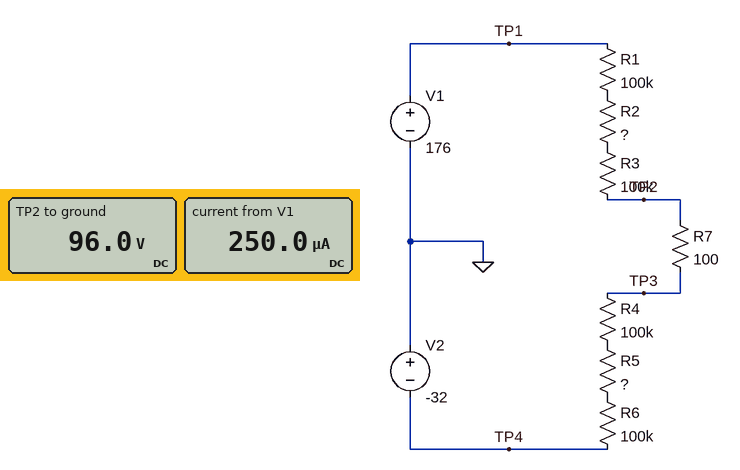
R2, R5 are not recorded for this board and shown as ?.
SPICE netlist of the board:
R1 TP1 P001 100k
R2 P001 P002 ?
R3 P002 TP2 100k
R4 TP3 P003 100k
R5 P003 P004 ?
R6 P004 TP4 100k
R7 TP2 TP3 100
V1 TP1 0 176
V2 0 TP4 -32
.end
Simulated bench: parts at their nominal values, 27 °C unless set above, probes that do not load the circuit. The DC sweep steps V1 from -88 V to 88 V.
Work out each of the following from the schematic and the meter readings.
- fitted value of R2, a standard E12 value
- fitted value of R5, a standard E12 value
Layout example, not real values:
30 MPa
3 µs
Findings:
120 kΩ
56 kΩ
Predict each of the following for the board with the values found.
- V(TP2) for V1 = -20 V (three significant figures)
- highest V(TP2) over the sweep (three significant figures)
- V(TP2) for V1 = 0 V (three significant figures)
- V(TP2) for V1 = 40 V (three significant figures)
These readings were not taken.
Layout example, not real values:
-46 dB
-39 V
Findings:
8.88 V
56.9 V
17.8 V
35.6 V
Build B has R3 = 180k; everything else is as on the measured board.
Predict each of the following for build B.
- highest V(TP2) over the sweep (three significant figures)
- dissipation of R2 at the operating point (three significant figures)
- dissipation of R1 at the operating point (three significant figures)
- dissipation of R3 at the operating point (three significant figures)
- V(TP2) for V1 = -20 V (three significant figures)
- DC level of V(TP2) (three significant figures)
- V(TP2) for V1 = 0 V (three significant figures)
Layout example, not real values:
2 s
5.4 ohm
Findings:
53.9 V
5.78 mW
4.82 mW
8.67 mW
11.7 V
88.2 V
19.5 V
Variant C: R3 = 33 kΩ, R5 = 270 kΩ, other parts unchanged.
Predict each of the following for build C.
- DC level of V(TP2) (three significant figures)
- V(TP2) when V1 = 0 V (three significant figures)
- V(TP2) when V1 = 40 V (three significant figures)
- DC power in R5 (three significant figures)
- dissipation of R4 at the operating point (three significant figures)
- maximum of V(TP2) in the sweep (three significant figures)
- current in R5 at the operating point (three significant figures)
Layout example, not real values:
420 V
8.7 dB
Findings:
126 V
11.2 V
37.2 V
10.7 mW
3.97 mW
68.4 V
199 µA
